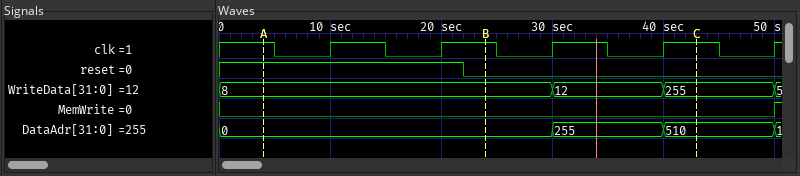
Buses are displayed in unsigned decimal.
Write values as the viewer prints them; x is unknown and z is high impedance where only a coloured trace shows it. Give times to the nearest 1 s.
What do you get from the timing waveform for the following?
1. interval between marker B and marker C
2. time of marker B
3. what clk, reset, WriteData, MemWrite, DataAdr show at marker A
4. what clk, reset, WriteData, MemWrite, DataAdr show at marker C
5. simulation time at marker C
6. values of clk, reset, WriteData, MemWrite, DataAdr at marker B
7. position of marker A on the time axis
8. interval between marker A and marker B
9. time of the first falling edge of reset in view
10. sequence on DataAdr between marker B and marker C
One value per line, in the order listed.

19 s
24 s
clk=1, reset=1, WriteData=8, MemWrite=0, DataAdr=0
clk=1, reset=0, WriteData=255, MemWrite=0, DataAdr=510
43 s
clk=1, reset=0, WriteData=8, MemWrite=0, DataAdr=0
4 s
20 s
22 s
0, 255, 510
